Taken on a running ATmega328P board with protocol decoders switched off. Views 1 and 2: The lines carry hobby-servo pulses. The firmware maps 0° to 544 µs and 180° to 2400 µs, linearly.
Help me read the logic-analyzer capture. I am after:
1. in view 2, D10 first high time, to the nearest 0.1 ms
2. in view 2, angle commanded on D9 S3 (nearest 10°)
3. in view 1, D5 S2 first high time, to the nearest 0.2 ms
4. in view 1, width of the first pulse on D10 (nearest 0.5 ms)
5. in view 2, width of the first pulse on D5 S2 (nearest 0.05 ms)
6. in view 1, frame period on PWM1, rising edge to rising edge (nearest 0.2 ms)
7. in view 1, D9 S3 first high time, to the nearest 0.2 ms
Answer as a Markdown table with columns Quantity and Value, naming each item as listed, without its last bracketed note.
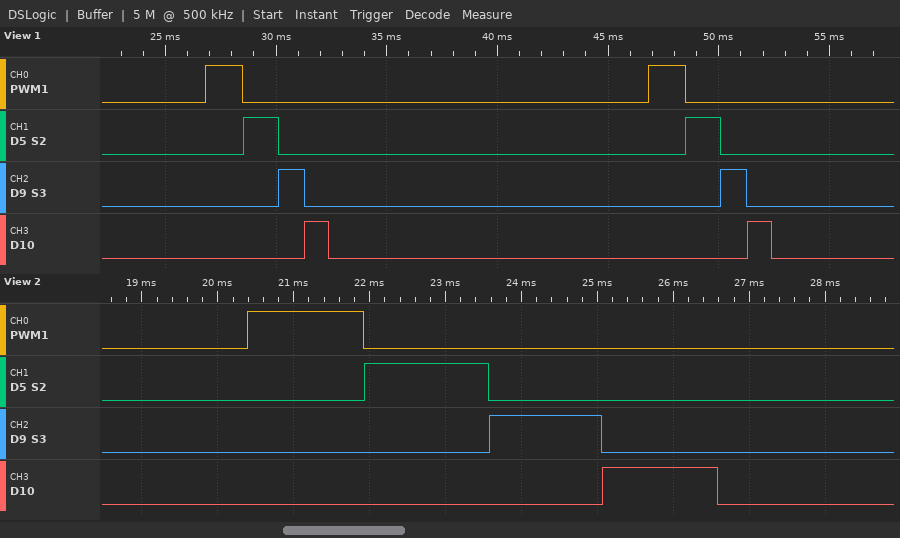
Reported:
| Quantity | Value |
|---|---|
| in view 2, D10 first high time, to the nearest 0.1 ms | 1.5 ms |
| in view 2, angle commanded on D9 S3 | 90° |
| in view 1, D5 S2 first high time, to the nearest 0.2 ms | 1.6 ms |
| in view 1, width of the first pulse on D10 | 1.0 ms |
| in view 2, width of the first pulse on D5 S2 | 1.65 ms |
| in view 1, frame period on PWM1, rising edge to rising edge | 20.0 ms |
| in view 1, D9 S3 first high time, to the nearest 0.2 ms | 1.2 ms |
